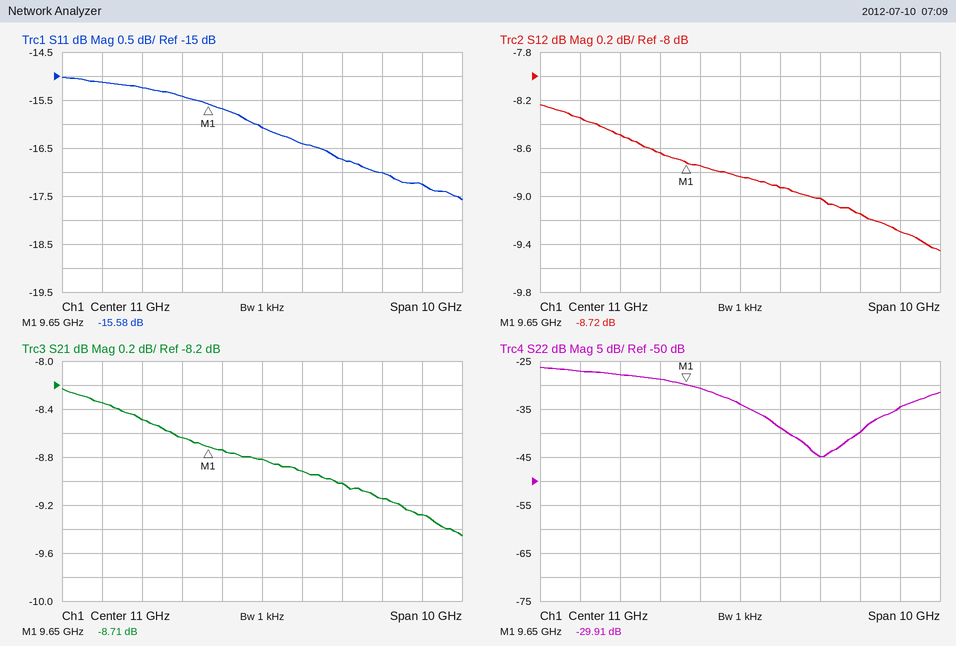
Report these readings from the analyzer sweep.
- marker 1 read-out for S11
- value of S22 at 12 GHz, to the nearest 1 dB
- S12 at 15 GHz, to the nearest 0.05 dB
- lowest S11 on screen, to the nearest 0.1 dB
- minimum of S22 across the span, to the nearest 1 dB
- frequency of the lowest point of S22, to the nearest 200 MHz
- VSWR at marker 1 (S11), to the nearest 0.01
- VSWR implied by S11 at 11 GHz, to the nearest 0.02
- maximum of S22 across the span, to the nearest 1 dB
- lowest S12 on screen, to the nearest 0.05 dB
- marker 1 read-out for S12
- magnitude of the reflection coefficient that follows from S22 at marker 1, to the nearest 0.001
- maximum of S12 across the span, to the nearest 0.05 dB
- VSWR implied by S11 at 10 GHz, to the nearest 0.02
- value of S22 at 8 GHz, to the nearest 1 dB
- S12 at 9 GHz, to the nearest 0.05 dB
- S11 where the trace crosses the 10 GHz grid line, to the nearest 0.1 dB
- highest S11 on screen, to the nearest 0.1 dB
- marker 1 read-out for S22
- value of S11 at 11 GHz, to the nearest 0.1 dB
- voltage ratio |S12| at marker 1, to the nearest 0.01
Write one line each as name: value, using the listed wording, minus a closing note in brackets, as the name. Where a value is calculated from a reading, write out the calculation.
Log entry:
marker 1 read-out for S11: -15.58 dB
value of S22 at 12 GHz, to the nearest 1 dB: -39 dB
S12 at 15 GHz, to the nearest 0.05 dB: -9.30 dB
lowest S11 on screen, to the nearest 0.1 dB: -17.6 dB
minimum of S22 across the span, to the nearest 1 dB: -45 dB
frequency of the lowest point of S22, to the nearest 200 MHz: 13.0 GHz
VSWR at marker 1 (S11), to the nearest 0.01: (1 + 0.1663)/(1 − 0.1663) ≈ 1.40
VSWR implied by S11 at 11 GHz, to the nearest 0.02: |Γ| = 10^(-16.1/20) = 0.1567; VSWR = (1 + 0.1567)/(1 − 0.1567) ≈ 1.37, so 1.38 to the nearest 0.02
maximum of S22 across the span, to the nearest 1 dB: -26 dB
lowest S12 on screen, to the nearest 0.05 dB: -9.45 dB
marker 1 read-out for S12: -8.72 dB
magnitude of the reflection coefficient that follows from S22 at marker 1, to the nearest 0.001: 10^(-29.91/20) ≈ 0.032
maximum of S12 across the span, to the nearest 0.05 dB: -8.25 dB
VSWR implied by S11 at 10 GHz, to the nearest 0.02: |Γ| = 10^(-15.7/20) = 0.1641; VSWR = (1 + 0.1641)/(1 − 0.1641) ≈ 1.39, so 1.40 to the nearest 0.02
value of S22 at 8 GHz, to the nearest 1 dB: -28 dB
S12 at 9 GHz, to the nearest 0.05 dB: -8.65 dB
S11 where the trace crosses the 10 GHz grid line, to the nearest 0.1 dB: -15.7 dB
highest S11 on screen, to the nearest 0.1 dB: -15.0 dB
marker 1 read-out for S22: -29.91 dB
value of S11 at 11 GHz, to the nearest 0.1 dB: -16.1 dB
voltage ratio |S12| at marker 1, to the nearest 0.01: 10^(-8.72/20) ≈ 0.37
